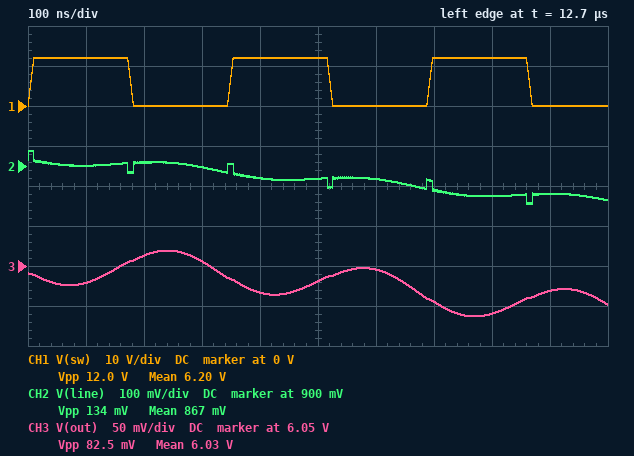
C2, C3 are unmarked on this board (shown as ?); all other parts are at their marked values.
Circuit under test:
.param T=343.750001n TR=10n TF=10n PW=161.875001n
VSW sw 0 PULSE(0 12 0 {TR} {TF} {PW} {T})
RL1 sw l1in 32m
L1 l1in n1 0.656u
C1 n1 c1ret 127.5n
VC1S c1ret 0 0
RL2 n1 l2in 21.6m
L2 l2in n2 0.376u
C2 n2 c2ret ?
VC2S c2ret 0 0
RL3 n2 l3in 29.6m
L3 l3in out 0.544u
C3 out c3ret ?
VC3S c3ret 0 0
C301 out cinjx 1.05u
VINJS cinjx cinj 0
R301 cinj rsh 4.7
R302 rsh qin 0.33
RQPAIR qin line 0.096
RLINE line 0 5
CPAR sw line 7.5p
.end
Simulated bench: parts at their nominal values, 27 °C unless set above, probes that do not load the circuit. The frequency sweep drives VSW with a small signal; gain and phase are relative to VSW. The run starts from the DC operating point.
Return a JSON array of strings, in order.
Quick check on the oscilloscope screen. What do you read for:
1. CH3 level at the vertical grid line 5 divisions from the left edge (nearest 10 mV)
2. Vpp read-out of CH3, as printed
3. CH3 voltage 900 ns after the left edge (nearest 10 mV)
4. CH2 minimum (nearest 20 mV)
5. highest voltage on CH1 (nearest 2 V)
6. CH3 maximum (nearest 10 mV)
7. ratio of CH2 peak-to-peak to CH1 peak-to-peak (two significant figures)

["6.03 V", "82.5 mV", "6.02 V", "800 mV", "12 V", "6.07 V", "0.011"]
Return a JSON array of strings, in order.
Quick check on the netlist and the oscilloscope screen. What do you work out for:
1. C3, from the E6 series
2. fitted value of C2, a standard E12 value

["22 nF", "47 nF"]
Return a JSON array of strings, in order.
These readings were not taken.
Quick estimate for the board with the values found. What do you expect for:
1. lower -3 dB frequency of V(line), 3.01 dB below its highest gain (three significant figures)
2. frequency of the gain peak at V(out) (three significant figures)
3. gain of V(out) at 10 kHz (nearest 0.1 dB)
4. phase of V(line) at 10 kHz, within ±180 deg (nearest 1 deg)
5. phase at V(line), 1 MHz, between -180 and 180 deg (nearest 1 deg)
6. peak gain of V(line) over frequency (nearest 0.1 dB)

["358 kHz", "426 kHz", "0 dB", "56 deg", "137 deg", "6.0 dB"]
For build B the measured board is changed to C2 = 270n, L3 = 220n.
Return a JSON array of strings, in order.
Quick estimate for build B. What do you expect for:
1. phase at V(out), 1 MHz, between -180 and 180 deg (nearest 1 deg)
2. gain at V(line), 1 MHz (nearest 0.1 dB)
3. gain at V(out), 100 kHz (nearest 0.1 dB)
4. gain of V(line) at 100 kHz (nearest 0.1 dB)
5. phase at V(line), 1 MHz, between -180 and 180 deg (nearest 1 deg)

["60 deg", "5.1 dB", "1.4 dB", "-4.8 dB", "61 deg"]
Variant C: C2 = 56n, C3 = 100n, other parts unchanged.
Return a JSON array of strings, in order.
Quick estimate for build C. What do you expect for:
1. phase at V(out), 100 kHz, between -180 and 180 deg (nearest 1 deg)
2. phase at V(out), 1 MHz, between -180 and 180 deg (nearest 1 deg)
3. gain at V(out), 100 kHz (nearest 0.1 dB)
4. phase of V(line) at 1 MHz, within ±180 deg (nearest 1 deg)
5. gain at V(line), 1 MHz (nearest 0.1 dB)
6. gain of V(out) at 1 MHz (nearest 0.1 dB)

["-7 deg", "16 deg", "1.1 dB", "17 deg", "-15.8 dB", "-9.7 dB"]
